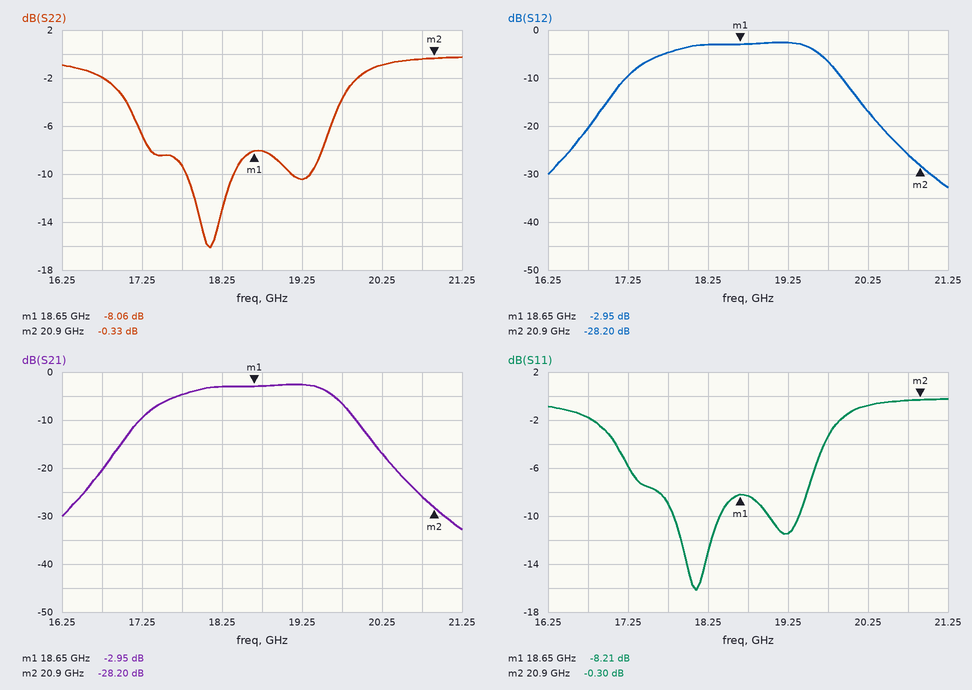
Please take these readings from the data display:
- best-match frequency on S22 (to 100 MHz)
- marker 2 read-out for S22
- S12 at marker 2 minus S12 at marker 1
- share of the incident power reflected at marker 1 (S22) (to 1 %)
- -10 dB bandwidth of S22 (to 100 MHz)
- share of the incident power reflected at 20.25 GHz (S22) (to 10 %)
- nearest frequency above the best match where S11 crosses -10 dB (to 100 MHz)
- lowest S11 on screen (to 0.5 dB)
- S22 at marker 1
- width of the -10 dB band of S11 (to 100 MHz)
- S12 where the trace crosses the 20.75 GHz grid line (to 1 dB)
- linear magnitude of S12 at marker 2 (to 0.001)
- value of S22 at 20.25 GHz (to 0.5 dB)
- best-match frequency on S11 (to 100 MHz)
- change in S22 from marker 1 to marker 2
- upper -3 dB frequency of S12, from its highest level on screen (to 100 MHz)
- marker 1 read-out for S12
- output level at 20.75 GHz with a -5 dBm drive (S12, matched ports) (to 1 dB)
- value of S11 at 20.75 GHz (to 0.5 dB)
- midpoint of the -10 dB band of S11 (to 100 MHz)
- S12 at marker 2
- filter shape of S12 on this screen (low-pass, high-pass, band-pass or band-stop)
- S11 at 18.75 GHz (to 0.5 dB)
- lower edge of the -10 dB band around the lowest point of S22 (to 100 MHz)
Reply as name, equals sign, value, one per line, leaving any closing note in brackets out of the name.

best-match frequency on S22 = 18.1 GHz
marker 2 read-out for S22 = -0.33 dB
S12 at marker 2 minus S12 at marker 1 = -25.25 dB
share of the incident power reflected at marker 1 (S22) = 16 %
-10 dB bandwidth of S22 = 600 MHz
share of the incident power reflected at 20.25 GHz (S22) = 80 %
nearest frequency above the best match where S11 crosses -10 dB = 18.4 GHz
lowest S11 on screen = -16.0 dB
S22 at marker 1 = -8.06 dB
width of the -10 dB band of S11 = 600 MHz
S12 where the trace crosses the 20.75 GHz grid line = -26 dB
linear magnitude of S12 at marker 2 = 0.039
value of S22 at 20.25 GHz = -1.0 dB
best-match frequency on S11 = 18.1 GHz
change in S22 from marker 1 to marker 2 = 7.73 dB
upper -3 dB frequency of S12, from its highest level on screen = 19.7 GHz
marker 1 read-out for S12 = -2.95 dB
output level at 20.75 GHz with a -5 dBm drive (S12, matched ports) = -31 dBm
value of S11 at 20.75 GHz = -0.5 dB
midpoint of the -10 dB band of S11 = 18.1 GHz
S12 at marker 2 = -28.20 dB
filter shape of S12 on this screen = band-pass
S11 at 18.75 GHz = -8.5 dB
lower edge of the -10 dB band around the lowest point of S22 = 17.8 GHz
